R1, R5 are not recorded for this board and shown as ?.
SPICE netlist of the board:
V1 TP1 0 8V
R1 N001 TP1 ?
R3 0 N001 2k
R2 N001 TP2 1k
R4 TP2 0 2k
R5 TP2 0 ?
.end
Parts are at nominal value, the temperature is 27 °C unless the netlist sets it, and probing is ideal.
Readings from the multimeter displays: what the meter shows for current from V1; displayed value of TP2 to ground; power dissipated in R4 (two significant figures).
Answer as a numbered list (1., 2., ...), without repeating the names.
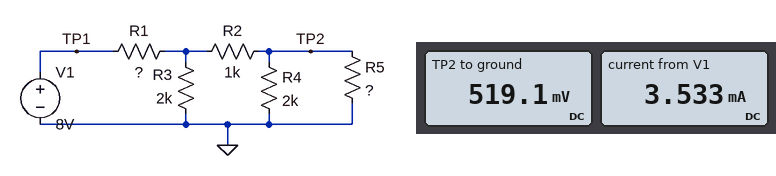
1. 3.533 mA
2. 519.1 mV
3. 130 µW
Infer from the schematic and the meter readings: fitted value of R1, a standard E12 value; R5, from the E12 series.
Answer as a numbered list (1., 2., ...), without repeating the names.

1. 1.5 kΩ
2. 270 Ω
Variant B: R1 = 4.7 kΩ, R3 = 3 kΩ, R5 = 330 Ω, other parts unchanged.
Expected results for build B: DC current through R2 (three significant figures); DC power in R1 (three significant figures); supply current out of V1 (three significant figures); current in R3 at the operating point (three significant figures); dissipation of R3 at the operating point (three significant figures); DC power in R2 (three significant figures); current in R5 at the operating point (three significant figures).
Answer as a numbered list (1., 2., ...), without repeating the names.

1. 1.00 mA
2. 9.60 mW
3. 1.43 mA
4. 428 µA
5. 550 µW
6. 1.00 mW
7. 859 µA
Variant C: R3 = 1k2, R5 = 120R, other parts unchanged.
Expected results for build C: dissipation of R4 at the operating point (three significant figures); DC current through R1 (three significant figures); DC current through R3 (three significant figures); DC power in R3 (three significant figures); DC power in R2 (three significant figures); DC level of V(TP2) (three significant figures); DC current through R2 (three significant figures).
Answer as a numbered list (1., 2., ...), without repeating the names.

1. 25.6 µW
2. 3.85 mA
3. 1.85 mA
4. 4.12 mW
5. 3.99 mW
6. 226 mV
7. 2.00 mA
